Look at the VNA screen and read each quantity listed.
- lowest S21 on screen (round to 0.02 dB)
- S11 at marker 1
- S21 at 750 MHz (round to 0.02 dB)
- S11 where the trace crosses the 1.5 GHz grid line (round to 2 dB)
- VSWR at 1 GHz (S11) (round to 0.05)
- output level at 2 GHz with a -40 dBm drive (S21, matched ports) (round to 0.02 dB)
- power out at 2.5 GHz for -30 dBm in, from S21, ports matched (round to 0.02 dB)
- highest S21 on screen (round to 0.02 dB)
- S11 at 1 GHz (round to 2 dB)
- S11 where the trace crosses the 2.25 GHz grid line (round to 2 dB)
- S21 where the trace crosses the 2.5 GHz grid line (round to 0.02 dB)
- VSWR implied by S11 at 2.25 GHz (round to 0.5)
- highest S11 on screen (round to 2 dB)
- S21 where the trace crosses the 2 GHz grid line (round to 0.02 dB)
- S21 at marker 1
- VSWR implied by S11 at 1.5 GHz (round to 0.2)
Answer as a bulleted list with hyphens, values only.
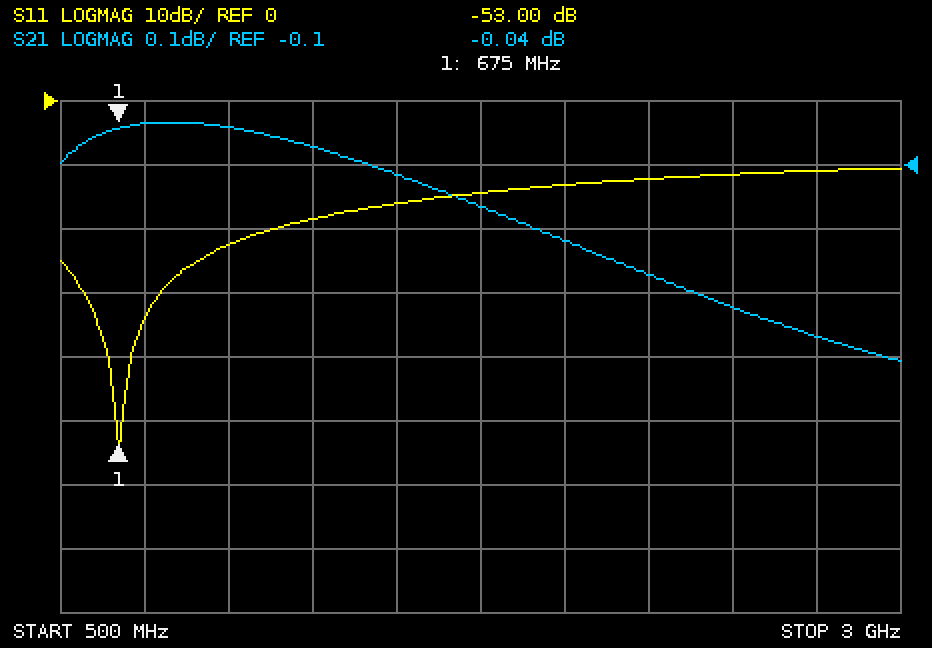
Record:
- -0.40 dB
- -53.00 dB
- -0.04 dB
- -16 dB
- 1.15
- -40.22 dBm
- -30.32 dBm
- -0.04 dB
- -22 dB
- -12 dB
- -0.32 dB
- 1.5
- -10 dB
- -0.22 dB
- -0.04 dB
- 1.4
